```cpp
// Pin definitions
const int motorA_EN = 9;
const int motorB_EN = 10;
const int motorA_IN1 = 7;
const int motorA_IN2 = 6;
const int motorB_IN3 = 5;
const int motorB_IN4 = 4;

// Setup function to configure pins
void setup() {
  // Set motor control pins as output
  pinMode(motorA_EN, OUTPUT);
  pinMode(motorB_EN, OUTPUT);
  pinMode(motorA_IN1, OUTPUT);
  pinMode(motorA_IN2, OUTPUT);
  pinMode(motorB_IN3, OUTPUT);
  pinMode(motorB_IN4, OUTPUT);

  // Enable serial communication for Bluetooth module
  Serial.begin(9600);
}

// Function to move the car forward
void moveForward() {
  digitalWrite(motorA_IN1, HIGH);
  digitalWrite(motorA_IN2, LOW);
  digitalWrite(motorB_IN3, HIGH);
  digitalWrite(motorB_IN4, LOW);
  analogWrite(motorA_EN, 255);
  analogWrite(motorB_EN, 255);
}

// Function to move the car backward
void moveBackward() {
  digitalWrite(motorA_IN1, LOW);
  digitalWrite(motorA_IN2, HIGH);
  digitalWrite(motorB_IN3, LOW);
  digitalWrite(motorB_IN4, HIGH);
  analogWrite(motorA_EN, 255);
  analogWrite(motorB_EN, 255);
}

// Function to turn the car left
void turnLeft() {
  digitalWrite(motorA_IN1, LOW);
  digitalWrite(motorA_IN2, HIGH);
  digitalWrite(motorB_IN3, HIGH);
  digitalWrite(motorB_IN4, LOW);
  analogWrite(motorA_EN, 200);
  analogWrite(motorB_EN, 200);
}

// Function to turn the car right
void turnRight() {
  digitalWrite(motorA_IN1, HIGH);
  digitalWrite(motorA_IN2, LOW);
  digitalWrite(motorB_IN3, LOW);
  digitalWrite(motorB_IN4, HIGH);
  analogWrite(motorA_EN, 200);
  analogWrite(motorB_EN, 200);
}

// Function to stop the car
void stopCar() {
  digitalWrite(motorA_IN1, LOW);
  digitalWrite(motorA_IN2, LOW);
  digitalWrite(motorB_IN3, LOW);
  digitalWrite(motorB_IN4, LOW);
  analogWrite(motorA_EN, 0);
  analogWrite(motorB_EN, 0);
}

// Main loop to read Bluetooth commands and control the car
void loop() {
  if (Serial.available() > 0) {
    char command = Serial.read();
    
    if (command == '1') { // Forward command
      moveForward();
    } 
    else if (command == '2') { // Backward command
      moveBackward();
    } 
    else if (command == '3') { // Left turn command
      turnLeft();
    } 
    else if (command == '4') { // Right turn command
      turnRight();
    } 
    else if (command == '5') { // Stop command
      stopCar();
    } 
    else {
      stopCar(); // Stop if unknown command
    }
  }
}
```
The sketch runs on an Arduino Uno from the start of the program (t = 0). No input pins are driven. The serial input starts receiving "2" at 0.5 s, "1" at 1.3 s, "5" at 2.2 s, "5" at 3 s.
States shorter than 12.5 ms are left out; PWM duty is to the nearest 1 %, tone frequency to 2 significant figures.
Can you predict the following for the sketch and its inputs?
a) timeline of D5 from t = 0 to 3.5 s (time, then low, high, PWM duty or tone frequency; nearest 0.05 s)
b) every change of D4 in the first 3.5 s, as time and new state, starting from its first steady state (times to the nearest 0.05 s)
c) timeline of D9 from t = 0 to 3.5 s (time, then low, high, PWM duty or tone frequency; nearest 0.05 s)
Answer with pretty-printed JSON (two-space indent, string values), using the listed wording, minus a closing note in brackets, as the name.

{
  "timeline of D5 from t = 0 to 3.5 s": "0 s low; 1.3 s high; 2.2 s low",
  "every change of D4 in the first 3.5 s, as time and new state, starting from its first steady state": "0 s low; 0.5 s high; 1.3 s low",
  "timeline of D9 from t = 0 to 3.5 s": "0 s low; 0.5 s high; 2.2 s low"
}
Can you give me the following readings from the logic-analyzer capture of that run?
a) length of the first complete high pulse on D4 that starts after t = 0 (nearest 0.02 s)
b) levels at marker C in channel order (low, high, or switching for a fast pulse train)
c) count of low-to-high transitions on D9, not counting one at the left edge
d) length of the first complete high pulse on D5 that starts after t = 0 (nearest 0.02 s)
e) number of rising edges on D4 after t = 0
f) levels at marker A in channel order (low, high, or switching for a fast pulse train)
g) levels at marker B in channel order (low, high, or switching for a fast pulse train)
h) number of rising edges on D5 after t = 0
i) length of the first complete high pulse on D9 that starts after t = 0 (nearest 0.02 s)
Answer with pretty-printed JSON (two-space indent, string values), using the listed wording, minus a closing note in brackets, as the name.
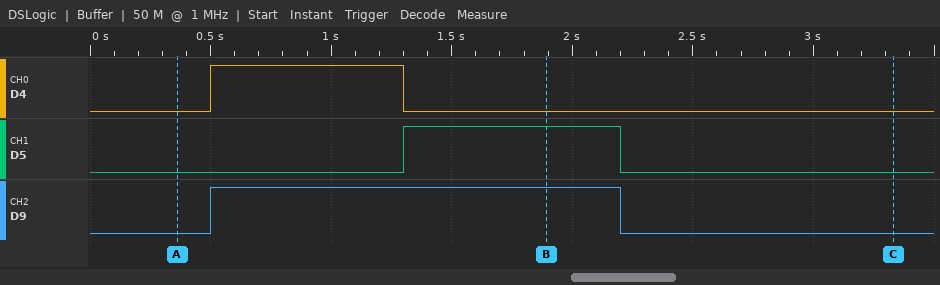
{
  "length of the first complete high pulse on D4 that starts after t = 0": "0.80 s",
  "levels at marker C in channel order": "D4 low, D5 low, D9 low",
  "count of low-to-high transitions on D9, not counting one at the left edge": "1",
  "length of the first complete high pulse on D5 that starts after t = 0": "0.90 s",
  "number of rising edges on D4 after t = 0": "1",
  "levels at marker A in channel order": "D4 low, D5 low, D9 low",
  "levels at marker B in channel order": "D4 low, D5 high, D9 high",
  "number of rising edges on D5 after t = 0": "1",
  "length of the first complete high pulse on D9 that starts after t = 0": "1.70 s"
}
